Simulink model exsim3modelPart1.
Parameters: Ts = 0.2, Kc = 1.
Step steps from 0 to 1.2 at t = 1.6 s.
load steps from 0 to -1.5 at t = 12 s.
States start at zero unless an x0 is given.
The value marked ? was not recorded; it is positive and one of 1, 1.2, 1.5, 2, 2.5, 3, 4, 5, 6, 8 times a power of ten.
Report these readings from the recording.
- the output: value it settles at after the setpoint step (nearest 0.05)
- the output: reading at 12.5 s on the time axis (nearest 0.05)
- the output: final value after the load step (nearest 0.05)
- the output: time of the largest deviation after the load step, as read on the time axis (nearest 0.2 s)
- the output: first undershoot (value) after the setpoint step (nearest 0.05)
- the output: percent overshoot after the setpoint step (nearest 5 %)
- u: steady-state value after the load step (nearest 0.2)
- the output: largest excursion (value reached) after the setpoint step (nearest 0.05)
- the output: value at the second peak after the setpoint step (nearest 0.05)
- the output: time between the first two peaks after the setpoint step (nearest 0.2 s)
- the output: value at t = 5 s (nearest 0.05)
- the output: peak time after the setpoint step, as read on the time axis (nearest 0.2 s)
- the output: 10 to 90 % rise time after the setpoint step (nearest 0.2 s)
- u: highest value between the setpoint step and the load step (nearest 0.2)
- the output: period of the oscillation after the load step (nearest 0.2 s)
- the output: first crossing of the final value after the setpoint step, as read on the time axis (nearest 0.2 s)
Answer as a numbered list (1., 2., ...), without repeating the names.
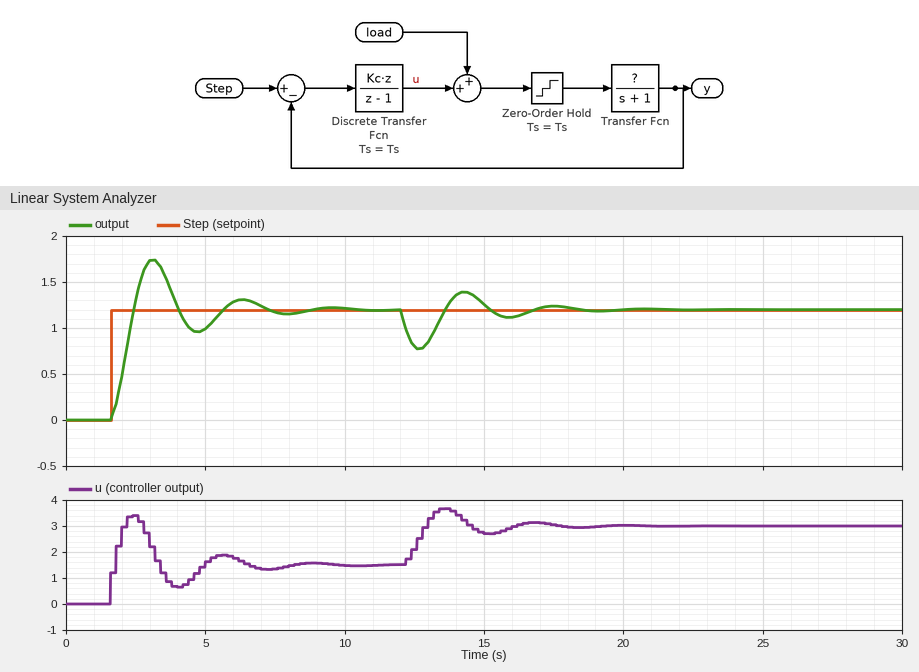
1. 1.20
2. 0.80
3. 1.20
4. 12.6 s
5. 0.95
6. 45 %
7. 3.0
8. 1.75
9. 1.30
10. 3.2 s
11. 1.00
12. 3.2 s
13. 0.6 s
14. 3.4
15. 3.2 s
16. 2.4 s
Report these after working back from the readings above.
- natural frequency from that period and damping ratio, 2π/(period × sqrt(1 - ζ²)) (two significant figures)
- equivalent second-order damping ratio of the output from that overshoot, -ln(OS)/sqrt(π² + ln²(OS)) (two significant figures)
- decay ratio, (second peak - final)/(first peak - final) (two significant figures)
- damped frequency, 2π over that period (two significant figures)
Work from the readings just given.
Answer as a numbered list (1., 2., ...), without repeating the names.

1. 2.0 rad/s
2. 0.25
3. 0.18
4. 2.0 rad/s
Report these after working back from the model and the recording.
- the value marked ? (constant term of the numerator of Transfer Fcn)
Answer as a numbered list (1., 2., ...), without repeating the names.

1. 0.8
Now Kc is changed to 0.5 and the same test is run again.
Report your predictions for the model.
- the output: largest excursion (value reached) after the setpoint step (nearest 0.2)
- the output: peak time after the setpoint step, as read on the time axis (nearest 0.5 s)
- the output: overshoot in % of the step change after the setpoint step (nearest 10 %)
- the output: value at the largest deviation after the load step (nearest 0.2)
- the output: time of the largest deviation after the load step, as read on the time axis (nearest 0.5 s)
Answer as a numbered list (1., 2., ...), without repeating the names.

1. 1.6
2. 4.0 s
3. 30 %
4. 0.6
5. 13.0 s
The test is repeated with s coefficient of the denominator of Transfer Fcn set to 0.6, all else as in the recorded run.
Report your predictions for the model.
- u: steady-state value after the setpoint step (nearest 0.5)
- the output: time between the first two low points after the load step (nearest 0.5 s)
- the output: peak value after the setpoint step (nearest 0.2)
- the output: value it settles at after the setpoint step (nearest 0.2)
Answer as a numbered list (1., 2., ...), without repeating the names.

1. 1.5
2. 2.5 s
3. 1.6
4. 1.2
